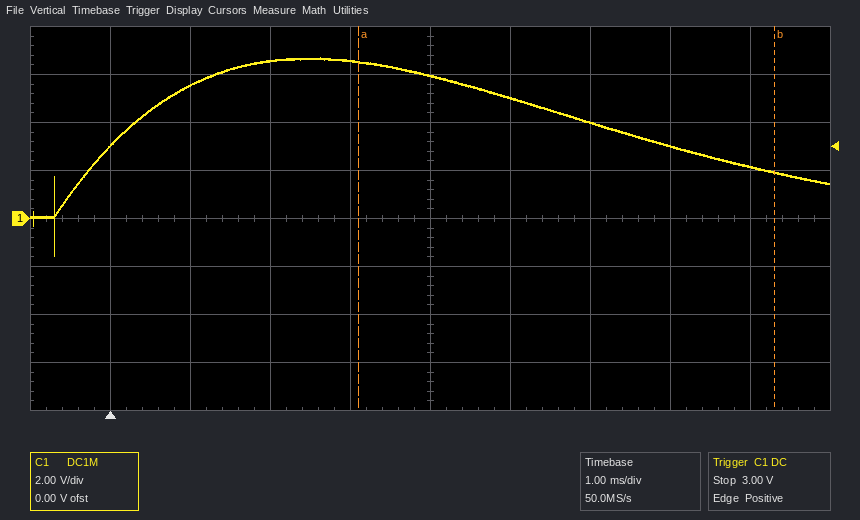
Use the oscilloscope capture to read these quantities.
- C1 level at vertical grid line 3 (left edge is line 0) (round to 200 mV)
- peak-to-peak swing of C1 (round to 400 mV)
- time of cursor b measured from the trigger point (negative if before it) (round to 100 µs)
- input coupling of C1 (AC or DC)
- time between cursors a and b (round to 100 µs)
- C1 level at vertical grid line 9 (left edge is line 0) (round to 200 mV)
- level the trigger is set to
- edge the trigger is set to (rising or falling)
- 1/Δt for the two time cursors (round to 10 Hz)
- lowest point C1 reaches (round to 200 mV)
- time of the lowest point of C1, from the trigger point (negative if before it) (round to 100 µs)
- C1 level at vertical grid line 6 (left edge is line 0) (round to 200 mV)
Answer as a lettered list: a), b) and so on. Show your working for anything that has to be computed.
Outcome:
a) 6.6 V
b) 8.4 V
c) +8.3 ms
d) DC
e) 5.2 ms
f) 2.2 V
g) 3.00 V
h) rising
i) 1 / 5.2 ms ≈ 190 Hz
j) -1.6 V
k) -700 µs
l) 5.0 V
